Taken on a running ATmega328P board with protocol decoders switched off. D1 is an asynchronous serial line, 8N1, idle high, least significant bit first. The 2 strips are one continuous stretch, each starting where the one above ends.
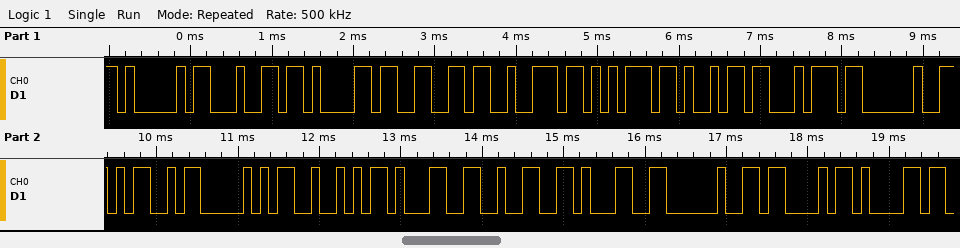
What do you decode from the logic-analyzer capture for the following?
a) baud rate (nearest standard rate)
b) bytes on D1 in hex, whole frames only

9600 baud
41 64 61 66 72 75 69 74 20 4D 50 52 31 32 31 20 43 61
